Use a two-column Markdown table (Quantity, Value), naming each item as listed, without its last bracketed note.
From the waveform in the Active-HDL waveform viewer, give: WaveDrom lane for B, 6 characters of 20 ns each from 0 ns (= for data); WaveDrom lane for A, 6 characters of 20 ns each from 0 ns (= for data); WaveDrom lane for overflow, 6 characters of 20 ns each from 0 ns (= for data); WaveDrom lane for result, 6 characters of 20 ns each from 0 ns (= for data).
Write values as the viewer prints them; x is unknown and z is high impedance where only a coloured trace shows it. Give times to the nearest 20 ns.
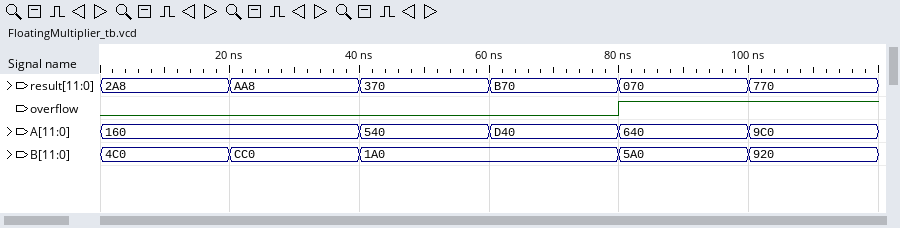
| Quantity | Value |
|---|---|
| WaveDrom lane for B, 6 characters of 20 ns each from 0 ns | {name: 'B', wave: '===.==', data: '4C0 CC0 1A0 5A0 920'} |
| WaveDrom lane for A, 6 characters of 20 ns each from 0 ns | {name: 'A', wave: '=.====', data: '160 540 D40 640 9C0'} |
| WaveDrom lane for overflow, 6 characters of 20 ns each from 0 ns | {name: 'overflow', wave: '0...1.'} |
| WaveDrom lane for result, 6 characters of 20 ns each from 0 ns | {name: 'result', wave: '======', data: '2A8 AA8 370 B70 070 770'} |
